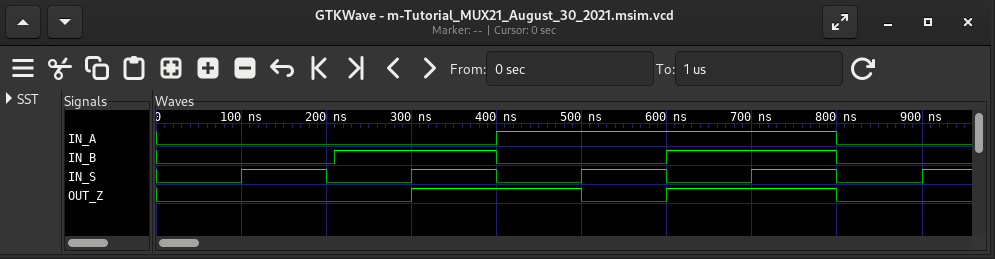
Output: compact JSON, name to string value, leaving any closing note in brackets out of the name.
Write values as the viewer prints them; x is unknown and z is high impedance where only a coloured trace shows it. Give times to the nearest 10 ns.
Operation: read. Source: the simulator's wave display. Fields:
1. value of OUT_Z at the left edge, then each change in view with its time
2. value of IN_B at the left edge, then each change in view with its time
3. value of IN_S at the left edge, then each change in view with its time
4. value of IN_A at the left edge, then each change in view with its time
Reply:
{"value of OUT_Z at the left edge, then each change in view with its time": "0, 1 at 300 ns, 0 at 500 ns, 1 at 600 ns, 0 at 800 ns", "value of IN_B at the left edge, then each change in view with its time": "0, 1 at 210 ns, 0 at 400 ns, 1 at 600 ns, 0 at 800 ns", "value of IN_S at the left edge, then each change in view with its time": "0, 1 at 100 ns, 0 at 200 ns, 1 at 300 ns, 0 at 400 ns, 1 at 500 ns, 0 at 600 ns, 1 at 700 ns, 0 at 800 ns, 1 at 900 ns", "value of IN_A at the left edge, then each change in view with its time": "0, 1 at 400 ns, 0 at 800 ns"}
